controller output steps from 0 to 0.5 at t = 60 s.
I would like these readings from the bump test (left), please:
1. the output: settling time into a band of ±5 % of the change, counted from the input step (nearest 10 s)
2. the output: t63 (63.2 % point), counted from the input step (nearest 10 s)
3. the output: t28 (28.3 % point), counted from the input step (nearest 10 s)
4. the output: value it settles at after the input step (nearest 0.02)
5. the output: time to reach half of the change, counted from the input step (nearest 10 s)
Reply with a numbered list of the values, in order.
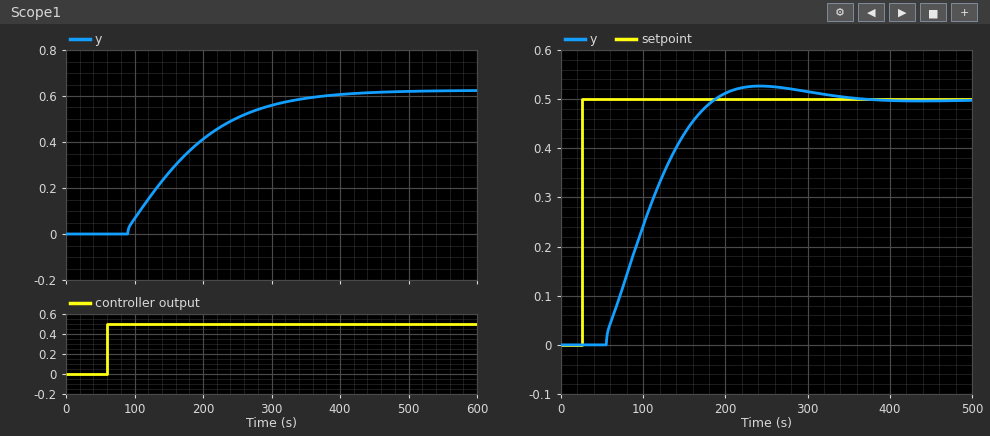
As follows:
1. 300 s
2. 130 s
3. 70 s
4. 0.62
5. 100 s
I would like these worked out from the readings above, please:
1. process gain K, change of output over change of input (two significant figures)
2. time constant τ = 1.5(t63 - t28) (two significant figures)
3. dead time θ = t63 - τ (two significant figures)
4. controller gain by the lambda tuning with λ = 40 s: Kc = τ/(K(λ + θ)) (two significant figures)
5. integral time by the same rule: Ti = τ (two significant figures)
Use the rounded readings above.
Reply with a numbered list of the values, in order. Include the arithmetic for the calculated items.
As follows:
1. (0.62 - 0) / 0.5 = 1.2
2. 1.5 × (130 - 70) = 90 s
3. 130 - 90 = 40 s
4. 90 / (1.2 × (40 + 40)) = 0.94
5. 90 s
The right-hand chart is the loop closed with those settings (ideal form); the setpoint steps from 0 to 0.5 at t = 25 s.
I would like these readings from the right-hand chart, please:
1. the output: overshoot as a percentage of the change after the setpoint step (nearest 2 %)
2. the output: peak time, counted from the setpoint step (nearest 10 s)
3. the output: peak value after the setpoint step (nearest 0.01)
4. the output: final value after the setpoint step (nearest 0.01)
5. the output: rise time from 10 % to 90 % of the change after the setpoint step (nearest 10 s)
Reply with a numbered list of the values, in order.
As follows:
1. 6 %
2. 220 s
3. 0.53
4. 0.50
5. 100 s
